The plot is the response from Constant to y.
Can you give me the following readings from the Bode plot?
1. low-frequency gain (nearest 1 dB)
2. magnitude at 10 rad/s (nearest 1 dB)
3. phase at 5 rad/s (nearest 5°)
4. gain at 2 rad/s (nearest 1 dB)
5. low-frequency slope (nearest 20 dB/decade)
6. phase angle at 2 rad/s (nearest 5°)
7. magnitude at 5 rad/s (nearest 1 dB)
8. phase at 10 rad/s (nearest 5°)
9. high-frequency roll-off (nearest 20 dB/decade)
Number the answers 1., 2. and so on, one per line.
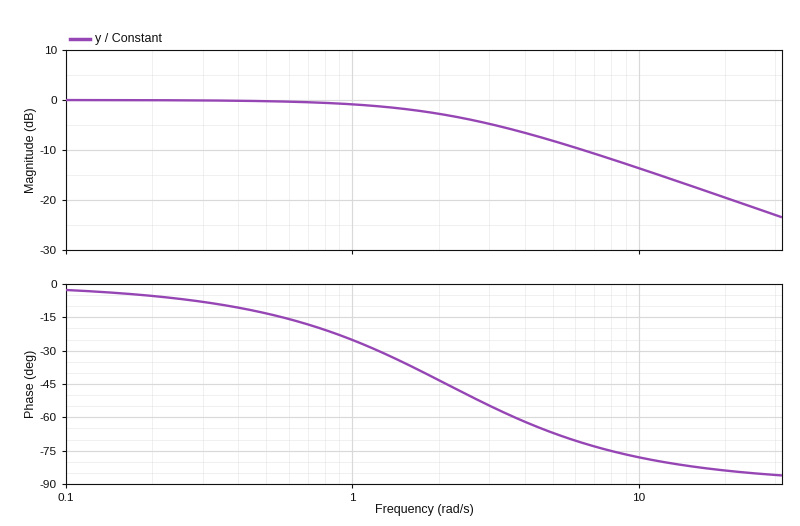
1. 0 dB
2. -14 dB
3. -65°
4. -3 dB
5. 0 dB/decade
6. -45°
7. -8 dB
8. -80°
9. -20 dB/decade
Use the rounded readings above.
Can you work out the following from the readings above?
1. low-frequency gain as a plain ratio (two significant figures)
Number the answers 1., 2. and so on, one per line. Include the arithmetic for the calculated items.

1. 10^(0 / 20) = 1.0
